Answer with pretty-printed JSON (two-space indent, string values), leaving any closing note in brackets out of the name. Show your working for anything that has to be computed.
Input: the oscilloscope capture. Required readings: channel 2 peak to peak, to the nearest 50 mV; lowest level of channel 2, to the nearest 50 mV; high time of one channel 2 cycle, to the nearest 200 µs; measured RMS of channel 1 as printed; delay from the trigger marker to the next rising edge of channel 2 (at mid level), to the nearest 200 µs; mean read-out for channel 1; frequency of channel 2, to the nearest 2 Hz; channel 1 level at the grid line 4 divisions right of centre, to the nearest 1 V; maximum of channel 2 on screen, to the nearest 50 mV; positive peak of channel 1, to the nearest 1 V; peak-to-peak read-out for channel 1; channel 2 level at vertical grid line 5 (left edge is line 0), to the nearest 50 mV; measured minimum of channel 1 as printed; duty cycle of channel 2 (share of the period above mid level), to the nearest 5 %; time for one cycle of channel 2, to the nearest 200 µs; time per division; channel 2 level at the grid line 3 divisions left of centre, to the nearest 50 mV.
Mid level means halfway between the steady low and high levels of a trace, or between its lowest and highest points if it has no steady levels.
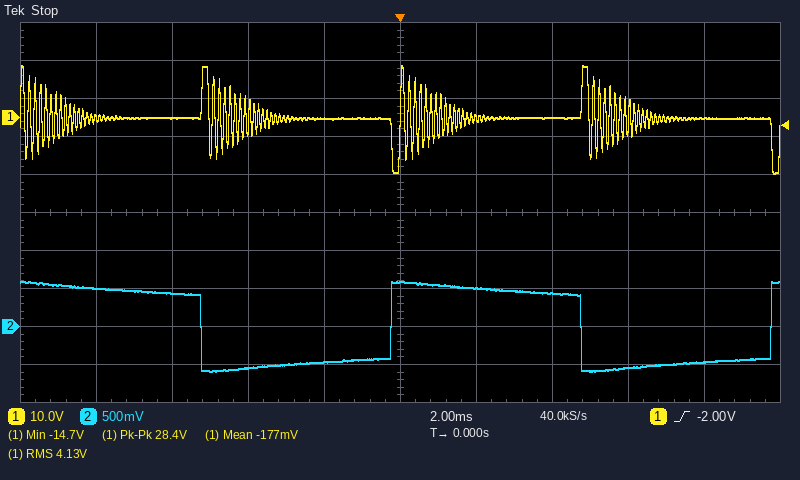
{
  "channel 2 peak to peak, to the nearest 50 mV": "600 mV − (-600 mV) = 1.20 V",
  "lowest level of channel 2, to the nearest 50 mV": "-600 mV",
  "high time of one channel 2 cycle, to the nearest 200 µs": "5.0 ms",
  "measured RMS of channel 1 as printed": "4.13 V",
  "delay from the trigger marker to the next rising edge of channel 2 (at mid level), to the nearest 200 µs": "9.8 ms",
  "mean read-out for channel 1": "-177 mV",
  "frequency of channel 2, to the nearest 2 Hz": "1 / 10.0 ms ≈ 100 Hz",
  "channel 1 level at the grid line 4 divisions right of centre, to the nearest 1 V": "0 V",
  "maximum of channel 2 on screen, to the nearest 50 mV": "600 mV",
  "positive peak of channel 1, to the nearest 1 V": "14 V",
  "peak-to-peak read-out for channel 1": "28.4 V",
  "channel 2 level at vertical grid line 5 (left edge is line 0), to the nearest 50 mV": "600 mV",
  "measured minimum of channel 1 as printed": "-14.7 V",
  "duty cycle of channel 2 (share of the period above mid level), to the nearest 5 %": "5.0 ms / 10.0 ms ≈ 50 %",
  "time for one cycle of channel 2, to the nearest 200 µs": "10.0 ms",
  "time per division": "2 ms",
  "channel 2 level at the grid line 3 divisions left of centre, to the nearest 50 mV": "450 mV"
}
